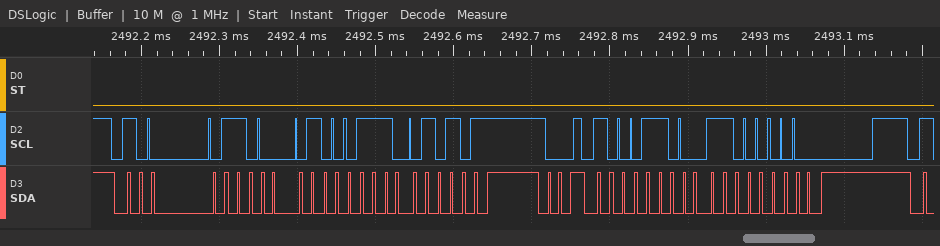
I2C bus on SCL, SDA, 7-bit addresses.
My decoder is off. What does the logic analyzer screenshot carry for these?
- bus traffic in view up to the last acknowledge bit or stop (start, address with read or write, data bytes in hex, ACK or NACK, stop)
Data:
start, address 46 write ACK, 47 ACK, 56 ACK, stop, start, address 46 write ACK, C0 ACK, stop
